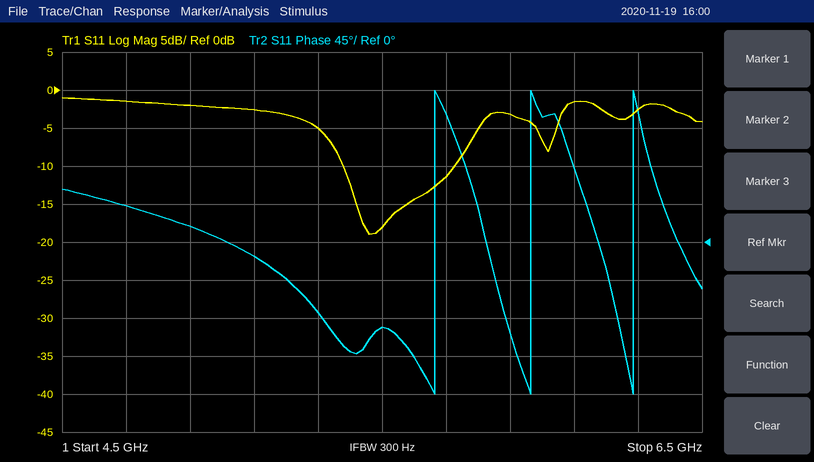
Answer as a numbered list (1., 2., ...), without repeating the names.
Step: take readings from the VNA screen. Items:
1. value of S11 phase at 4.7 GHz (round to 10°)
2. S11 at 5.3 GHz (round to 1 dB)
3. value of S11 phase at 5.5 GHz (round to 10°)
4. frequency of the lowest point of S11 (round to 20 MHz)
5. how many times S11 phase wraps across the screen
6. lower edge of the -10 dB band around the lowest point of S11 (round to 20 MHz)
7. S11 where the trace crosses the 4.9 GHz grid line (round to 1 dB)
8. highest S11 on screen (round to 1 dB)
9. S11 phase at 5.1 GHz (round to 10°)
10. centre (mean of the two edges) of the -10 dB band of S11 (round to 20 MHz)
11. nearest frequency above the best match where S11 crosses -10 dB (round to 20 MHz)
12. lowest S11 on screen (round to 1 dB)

1. 40°
2. -5 dB
3. -100°
4. 5.46 GHz
5. 3
6. 5.38 GHz
7. -2 dB
8. -1 dB
9. -20°
10. 5.56 GHz
11. 5.72 GHz
12. -19 dB
